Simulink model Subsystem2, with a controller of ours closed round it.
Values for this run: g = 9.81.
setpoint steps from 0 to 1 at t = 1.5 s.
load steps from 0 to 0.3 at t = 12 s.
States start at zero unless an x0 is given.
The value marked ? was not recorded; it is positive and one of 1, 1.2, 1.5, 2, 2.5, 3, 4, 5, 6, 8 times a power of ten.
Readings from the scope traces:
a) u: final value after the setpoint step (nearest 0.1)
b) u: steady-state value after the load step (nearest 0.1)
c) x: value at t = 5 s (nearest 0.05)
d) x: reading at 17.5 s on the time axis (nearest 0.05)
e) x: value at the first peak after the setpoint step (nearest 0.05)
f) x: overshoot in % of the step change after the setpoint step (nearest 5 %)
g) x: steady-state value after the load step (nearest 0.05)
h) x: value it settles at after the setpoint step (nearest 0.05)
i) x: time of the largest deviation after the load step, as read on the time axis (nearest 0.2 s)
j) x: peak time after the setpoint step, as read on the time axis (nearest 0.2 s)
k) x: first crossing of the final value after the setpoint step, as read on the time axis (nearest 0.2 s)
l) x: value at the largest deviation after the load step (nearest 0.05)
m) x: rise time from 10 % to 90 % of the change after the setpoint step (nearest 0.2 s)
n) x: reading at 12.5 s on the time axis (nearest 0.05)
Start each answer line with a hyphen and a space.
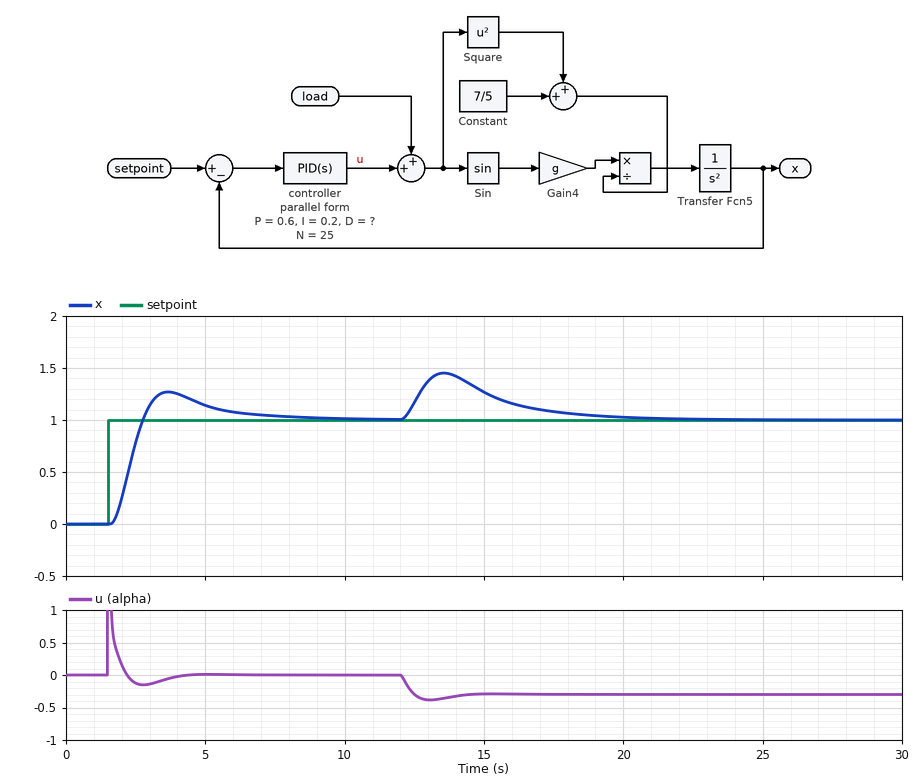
- 0.0
- -0.3
- 1.15
- 1.10
- 1.25
- 25 %
- 1.00
- 1.00
- 13.6 s
- 3.6 s
- 2.8 s
- 1.45
- 0.8 s
- 1.15
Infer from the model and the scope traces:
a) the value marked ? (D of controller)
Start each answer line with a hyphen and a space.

- 0.4
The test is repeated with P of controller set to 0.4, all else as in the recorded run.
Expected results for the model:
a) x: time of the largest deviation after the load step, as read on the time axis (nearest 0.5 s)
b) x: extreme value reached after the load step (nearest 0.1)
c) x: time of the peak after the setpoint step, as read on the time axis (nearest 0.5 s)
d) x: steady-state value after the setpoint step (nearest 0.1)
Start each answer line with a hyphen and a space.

- 14.0 s
- 1.6
- 4.5 s
- 1.0
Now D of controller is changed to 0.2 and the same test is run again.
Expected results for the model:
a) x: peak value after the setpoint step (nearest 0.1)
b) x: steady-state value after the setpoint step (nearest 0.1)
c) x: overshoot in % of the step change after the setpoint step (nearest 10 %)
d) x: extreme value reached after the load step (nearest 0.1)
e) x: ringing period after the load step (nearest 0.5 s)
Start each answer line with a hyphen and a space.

- 1.6
- 1.0
- 60 %
- 1.6
- 3.0 s
